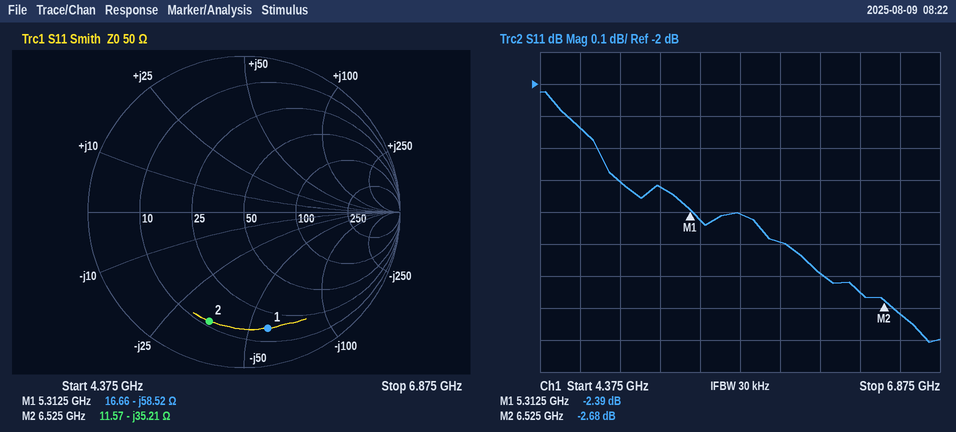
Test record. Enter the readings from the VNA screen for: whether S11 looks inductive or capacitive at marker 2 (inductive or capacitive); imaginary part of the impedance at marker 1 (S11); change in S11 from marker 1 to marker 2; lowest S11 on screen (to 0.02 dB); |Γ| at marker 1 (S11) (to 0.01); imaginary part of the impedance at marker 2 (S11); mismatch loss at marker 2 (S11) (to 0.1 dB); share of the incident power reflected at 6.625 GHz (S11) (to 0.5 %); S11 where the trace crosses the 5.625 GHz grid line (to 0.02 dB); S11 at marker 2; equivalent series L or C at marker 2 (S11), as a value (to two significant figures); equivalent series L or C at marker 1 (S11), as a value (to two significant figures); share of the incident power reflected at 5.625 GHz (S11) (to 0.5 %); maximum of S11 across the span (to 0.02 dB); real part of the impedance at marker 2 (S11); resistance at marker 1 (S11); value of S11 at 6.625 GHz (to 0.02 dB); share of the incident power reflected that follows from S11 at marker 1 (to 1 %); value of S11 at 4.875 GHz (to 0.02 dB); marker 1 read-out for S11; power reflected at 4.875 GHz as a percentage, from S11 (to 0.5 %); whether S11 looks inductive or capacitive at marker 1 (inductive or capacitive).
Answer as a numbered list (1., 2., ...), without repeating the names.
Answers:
1. capacitive
2. -58.52 Ω
3. -0.29 dB
4. -2.80 dB
5. 0.76
6. -35.21 Ω
7. 3.4 dB
8. 53.5 %
9. -2.40 dB
10. -2.68 dB
11. 690 fF
12. 510 fF
13. 57.5 %
14. -2.02 dB
15. 11.57 Ω
16. 16.66 Ω
17. -2.72 dB
18. 58 %
19. -2.30 dB
20. -2.39 dB
21. 59.0 %
22. capacitive
